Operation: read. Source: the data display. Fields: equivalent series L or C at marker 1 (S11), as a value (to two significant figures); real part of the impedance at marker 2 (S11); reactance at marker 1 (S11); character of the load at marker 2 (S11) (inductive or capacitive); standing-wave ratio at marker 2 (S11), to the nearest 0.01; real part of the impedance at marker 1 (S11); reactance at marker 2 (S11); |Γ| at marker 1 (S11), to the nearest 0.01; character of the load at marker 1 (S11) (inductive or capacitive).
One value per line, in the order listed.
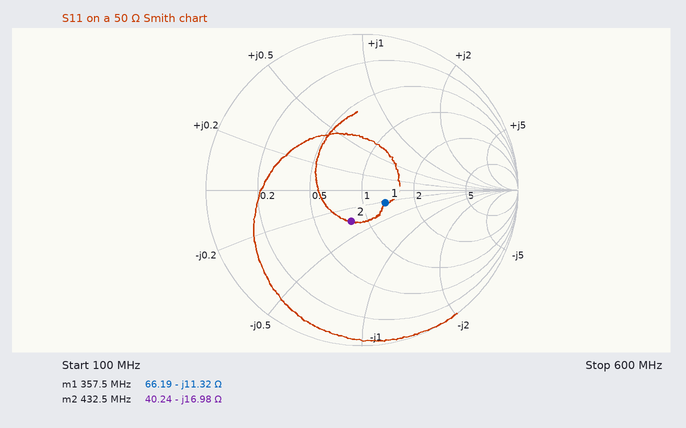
39 pF
40.24 Ω
-11.32 Ω
capacitive
1.54
66.19 Ω
-16.98 Ω
0.17
capacitive
